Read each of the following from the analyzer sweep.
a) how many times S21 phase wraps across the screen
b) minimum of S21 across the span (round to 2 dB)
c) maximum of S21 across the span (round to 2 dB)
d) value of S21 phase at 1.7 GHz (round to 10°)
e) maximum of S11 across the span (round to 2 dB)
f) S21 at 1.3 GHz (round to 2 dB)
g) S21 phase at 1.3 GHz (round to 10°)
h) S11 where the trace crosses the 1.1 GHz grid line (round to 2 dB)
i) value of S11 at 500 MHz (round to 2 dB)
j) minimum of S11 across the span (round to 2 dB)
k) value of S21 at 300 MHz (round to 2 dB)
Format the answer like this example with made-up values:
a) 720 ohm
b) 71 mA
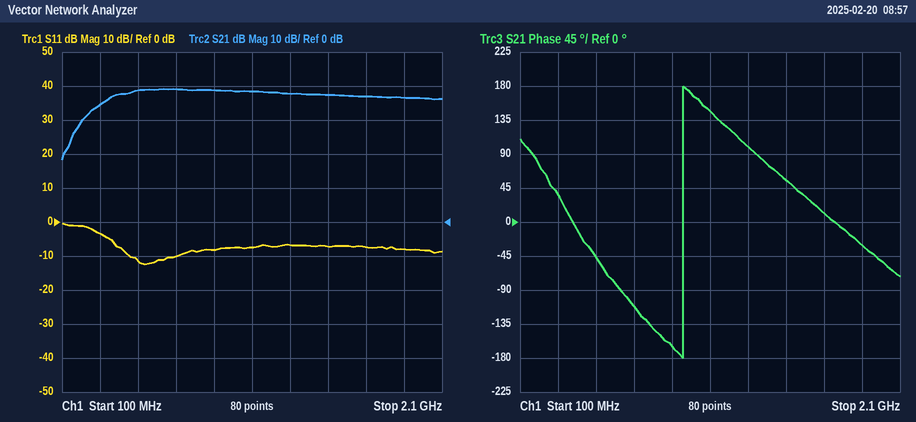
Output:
a) 1
b) 18 dB
c) 40 dB
d) 10°
e) 0 dB
f) 38 dB
g) 100°
h) -8 dB
i) -12 dB
j) -12 dB
k) 34 dB
